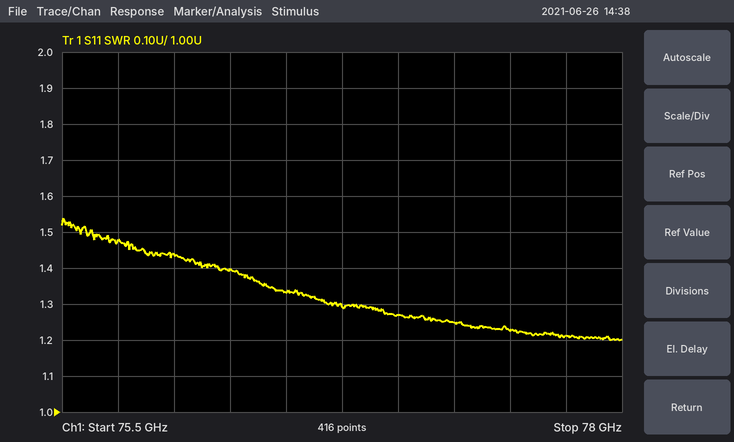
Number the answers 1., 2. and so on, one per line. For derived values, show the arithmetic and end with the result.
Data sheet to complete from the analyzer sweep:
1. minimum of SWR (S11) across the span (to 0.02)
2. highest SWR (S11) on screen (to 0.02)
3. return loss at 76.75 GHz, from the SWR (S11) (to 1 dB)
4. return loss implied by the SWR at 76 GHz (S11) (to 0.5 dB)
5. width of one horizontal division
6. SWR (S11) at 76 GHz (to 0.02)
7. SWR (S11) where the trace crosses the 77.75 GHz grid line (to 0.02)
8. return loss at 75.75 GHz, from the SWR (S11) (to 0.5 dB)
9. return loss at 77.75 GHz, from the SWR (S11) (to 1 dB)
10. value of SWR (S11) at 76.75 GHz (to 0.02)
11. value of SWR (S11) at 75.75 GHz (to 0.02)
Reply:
1. 1.20
2. 1.54
3. −20 log10((1.3 − 1)/(1.3 + 1)) ≈ 18 dB
4. −20 log10((1.44 − 1)/(1.44 + 1)) ≈ 14.9 dB, so 15.0 dB to the nearest 0.5 dB
5. 250 MHz
6. 1.44
7. 1.22
8. −20 log10((1.48 − 1)/(1.48 + 1)) ≈ 14.3 dB, so 14.5 dB to the nearest 0.5 dB
9. −20 log10((1.22 − 1)/(1.22 + 1)) ≈ 20 dB
10. 1.30
11. 1.48
